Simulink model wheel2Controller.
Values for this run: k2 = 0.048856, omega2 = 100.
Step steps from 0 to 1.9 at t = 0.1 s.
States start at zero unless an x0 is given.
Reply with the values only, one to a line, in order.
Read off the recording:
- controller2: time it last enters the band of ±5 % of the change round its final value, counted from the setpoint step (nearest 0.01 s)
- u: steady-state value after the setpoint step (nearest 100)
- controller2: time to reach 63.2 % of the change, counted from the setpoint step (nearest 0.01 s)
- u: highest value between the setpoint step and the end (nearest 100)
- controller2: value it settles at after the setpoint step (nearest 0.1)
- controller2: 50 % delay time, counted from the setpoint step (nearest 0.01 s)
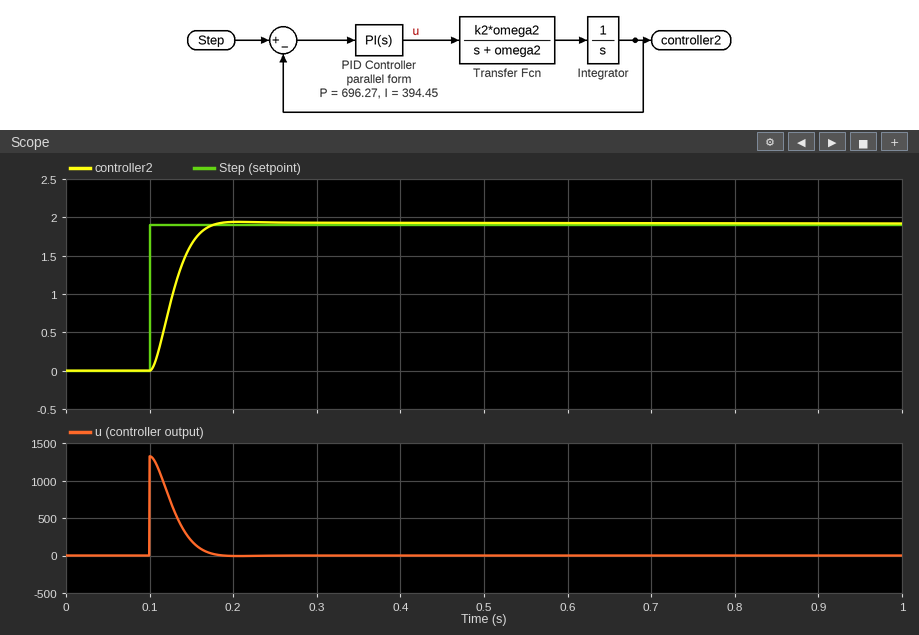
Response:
0.06 s
0
0.03 s
1300
1.9
0.03 s
